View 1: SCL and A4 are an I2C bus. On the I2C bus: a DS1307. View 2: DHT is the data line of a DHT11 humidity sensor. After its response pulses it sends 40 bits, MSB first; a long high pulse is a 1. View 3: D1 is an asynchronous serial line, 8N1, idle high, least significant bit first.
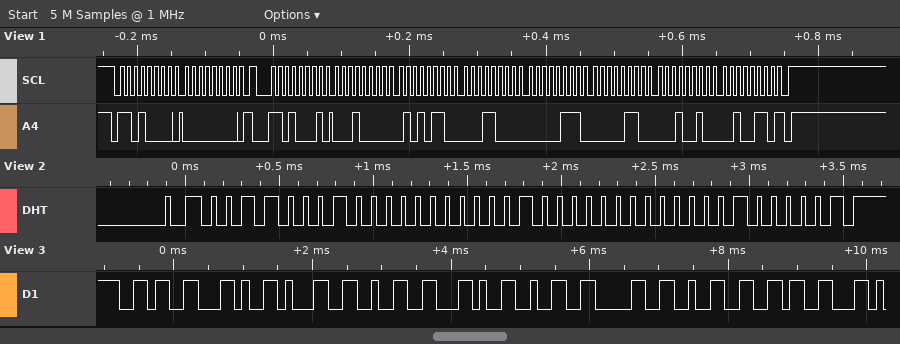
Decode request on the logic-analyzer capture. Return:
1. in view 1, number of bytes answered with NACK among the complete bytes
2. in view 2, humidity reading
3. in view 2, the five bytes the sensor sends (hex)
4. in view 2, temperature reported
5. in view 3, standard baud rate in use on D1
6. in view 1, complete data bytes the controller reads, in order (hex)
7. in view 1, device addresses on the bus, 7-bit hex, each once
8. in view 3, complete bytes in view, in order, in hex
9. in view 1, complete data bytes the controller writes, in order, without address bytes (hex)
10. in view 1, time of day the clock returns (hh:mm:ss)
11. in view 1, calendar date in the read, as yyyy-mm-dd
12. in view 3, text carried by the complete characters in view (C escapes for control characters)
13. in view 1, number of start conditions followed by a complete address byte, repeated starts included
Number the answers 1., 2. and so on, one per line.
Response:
1. 1
2. 49 %
3. 31 00 10 00 41
4. 16.0 °C
5. 9600 baud
6. 10 56 18 07 06 12 26
7. 0x68
8. 36 2C 31 32 2C 32 30 32 36
9. 00
10. 18:56:10
11. 2026-12-06
12. "6,12,2026"
13. 2
